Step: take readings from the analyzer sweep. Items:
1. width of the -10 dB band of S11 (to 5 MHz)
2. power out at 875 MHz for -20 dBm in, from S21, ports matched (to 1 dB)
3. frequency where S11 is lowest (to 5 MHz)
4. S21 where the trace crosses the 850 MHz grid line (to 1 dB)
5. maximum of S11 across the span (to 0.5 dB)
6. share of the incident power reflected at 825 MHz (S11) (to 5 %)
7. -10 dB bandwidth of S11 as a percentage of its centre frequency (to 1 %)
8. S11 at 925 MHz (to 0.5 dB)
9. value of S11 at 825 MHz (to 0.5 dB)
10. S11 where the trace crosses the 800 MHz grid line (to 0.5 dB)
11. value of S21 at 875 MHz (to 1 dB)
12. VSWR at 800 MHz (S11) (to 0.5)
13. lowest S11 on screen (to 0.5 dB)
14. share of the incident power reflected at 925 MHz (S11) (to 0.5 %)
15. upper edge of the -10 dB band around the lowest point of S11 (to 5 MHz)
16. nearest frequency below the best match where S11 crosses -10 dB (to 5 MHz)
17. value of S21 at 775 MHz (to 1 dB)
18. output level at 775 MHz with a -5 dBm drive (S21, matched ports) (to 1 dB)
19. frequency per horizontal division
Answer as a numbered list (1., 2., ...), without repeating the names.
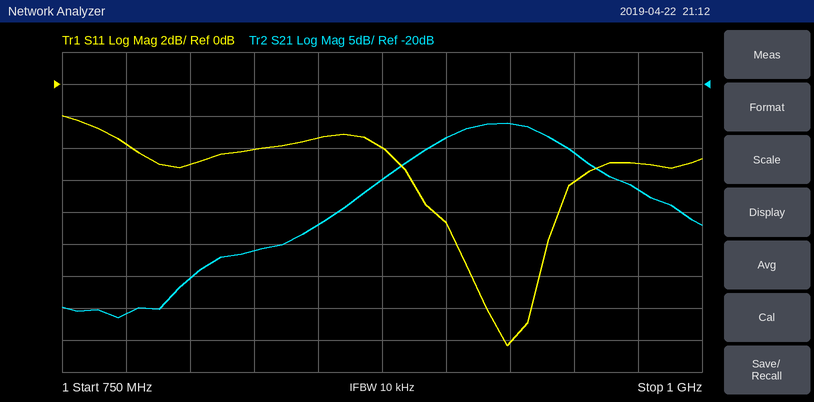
1. 35 MHz
2. -55 dBm
3. 925 MHz
4. -42 dB
5. -2.0 dB
6. 40 %
7. 4 %
8. -16.0 dB
9. -4.0 dB
10. -5.0 dB
11. -35 dB
12. 3.5
13. -16.5 dB
14. 2.5 %
15. 940 MHz
16. 905 MHz
17. -56 dB
18. -61 dBm
19. 25 MHz
